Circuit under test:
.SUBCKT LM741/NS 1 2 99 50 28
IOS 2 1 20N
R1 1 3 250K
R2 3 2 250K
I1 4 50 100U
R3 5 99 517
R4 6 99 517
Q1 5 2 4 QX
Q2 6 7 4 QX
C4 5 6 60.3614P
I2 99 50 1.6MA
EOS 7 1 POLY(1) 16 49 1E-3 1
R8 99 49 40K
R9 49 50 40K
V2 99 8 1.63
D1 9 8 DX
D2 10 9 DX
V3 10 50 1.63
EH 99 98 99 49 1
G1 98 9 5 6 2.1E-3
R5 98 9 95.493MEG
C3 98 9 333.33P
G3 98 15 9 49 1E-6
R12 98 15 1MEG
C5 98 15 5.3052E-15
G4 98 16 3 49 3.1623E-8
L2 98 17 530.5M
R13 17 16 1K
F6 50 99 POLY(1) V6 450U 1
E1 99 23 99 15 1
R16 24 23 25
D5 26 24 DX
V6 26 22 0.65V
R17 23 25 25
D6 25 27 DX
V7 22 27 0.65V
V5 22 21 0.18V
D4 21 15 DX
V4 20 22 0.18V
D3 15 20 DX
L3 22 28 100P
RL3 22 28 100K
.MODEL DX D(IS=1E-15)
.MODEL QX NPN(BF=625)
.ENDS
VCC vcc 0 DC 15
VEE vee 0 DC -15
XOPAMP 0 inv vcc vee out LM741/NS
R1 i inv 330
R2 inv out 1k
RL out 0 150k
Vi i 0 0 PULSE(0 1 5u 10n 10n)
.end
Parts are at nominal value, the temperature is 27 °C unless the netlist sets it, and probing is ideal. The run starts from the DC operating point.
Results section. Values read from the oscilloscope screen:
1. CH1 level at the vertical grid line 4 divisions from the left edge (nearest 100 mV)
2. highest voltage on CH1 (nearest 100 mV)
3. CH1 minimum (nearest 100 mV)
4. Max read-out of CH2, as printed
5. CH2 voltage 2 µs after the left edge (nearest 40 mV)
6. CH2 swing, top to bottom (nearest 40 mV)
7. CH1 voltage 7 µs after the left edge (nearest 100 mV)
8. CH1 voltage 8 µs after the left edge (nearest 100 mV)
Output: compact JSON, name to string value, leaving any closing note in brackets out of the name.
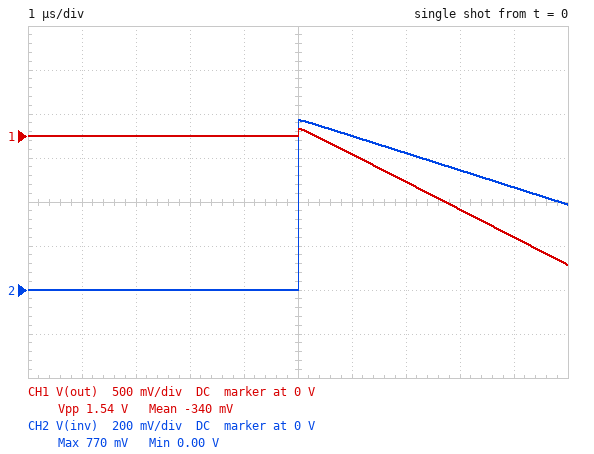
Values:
{"CH1 level at the vertical grid line 4 divisions from the left edge": "0 V", "highest voltage on CH1": "100 mV", "CH1 minimum": "-1.5 V", "Max read-out of CH2, as printed": "770 mV", "CH2 voltage 2 µs after the left edge": "0 V", "CH2 swing, top to bottom": "760 mV", "CH1 voltage 7 µs after the left edge": "-500 mV", "CH1 voltage 8 µs after the left edge": "-800 mV"}
